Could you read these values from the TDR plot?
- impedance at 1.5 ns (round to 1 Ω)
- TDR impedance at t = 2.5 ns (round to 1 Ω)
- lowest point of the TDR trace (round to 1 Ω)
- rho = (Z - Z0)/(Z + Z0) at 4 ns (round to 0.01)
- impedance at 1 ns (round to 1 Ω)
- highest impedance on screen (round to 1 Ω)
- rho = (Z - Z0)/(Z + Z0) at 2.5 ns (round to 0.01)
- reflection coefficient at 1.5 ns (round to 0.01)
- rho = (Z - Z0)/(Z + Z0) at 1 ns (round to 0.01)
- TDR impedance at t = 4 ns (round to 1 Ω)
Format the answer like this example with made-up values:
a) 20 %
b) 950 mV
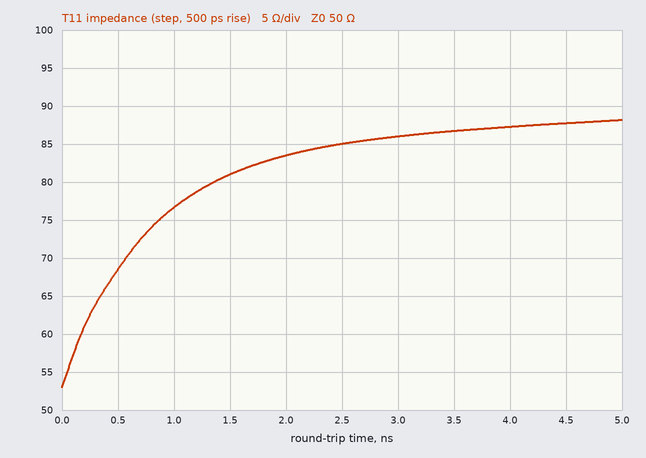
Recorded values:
a) 81 Ω
b) 85 Ω
c) 53 Ω
d) +0.27
e) 77 Ω
f) 88 Ω
g) +0.26
h) +0.24
i) +0.21
j) 87 Ω
